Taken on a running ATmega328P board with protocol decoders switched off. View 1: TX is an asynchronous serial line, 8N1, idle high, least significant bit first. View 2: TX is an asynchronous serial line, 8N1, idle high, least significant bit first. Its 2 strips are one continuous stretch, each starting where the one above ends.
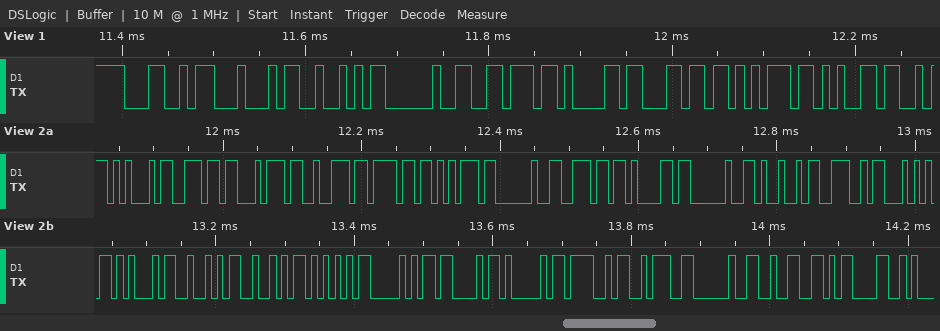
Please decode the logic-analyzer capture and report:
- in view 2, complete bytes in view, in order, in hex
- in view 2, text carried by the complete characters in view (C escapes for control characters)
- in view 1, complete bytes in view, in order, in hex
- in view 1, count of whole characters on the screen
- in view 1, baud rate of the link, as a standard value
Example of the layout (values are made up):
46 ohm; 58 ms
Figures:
45 6E 74 72 6F 75 20 6E 61 20 49 4E 54 45 52 52 55 50 43 41 4F 3A 20 32 0D; "Entrou na INTERRUPCAO: 2\r"; 4C 44 52 20 76 61 6C 75 65; 9; 115200 baud
